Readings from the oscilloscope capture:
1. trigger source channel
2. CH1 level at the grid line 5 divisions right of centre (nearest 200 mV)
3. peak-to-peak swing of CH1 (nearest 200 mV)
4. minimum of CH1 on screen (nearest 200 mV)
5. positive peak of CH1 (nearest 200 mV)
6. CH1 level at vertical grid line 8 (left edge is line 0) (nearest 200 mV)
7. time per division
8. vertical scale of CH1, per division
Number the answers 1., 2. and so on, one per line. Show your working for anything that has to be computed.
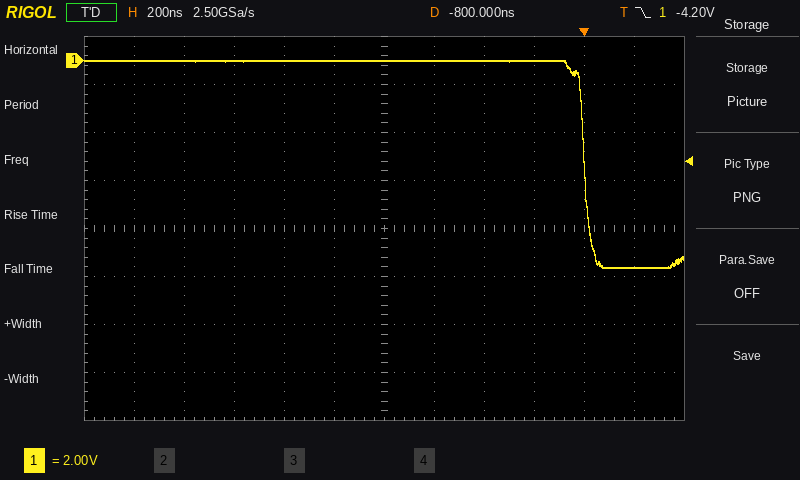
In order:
1. CH1
2. -8.6 V
3. 0.0 V − (-8.6 V) = 8.6 V
4. -8.6 V
5. 0.0 V
6. 0.0 V
7. 200 ns
8. 2 V
